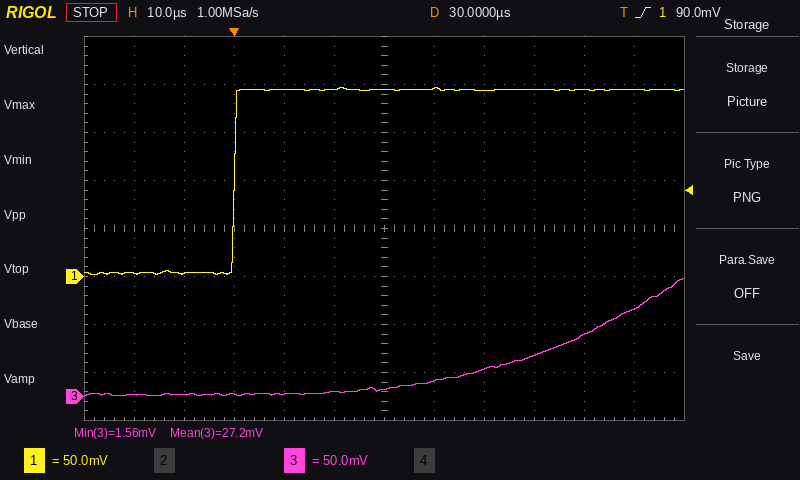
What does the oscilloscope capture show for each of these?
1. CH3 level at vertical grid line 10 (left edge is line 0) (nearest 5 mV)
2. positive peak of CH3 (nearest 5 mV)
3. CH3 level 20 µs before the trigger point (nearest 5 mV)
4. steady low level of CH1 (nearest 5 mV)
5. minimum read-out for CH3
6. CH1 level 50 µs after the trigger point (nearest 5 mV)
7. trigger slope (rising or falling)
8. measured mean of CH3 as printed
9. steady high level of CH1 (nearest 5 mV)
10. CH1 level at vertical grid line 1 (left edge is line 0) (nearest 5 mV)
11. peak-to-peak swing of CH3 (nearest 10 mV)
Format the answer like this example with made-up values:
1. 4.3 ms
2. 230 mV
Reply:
1. 65 mV
2. 125 mV
3. 0 mV
4. 5 mV
5. 1.56 mV
6. 195 mV
7. rising
8. 27.2 mV
9. 195 mV
10. 5 mV
11. 120 mV
